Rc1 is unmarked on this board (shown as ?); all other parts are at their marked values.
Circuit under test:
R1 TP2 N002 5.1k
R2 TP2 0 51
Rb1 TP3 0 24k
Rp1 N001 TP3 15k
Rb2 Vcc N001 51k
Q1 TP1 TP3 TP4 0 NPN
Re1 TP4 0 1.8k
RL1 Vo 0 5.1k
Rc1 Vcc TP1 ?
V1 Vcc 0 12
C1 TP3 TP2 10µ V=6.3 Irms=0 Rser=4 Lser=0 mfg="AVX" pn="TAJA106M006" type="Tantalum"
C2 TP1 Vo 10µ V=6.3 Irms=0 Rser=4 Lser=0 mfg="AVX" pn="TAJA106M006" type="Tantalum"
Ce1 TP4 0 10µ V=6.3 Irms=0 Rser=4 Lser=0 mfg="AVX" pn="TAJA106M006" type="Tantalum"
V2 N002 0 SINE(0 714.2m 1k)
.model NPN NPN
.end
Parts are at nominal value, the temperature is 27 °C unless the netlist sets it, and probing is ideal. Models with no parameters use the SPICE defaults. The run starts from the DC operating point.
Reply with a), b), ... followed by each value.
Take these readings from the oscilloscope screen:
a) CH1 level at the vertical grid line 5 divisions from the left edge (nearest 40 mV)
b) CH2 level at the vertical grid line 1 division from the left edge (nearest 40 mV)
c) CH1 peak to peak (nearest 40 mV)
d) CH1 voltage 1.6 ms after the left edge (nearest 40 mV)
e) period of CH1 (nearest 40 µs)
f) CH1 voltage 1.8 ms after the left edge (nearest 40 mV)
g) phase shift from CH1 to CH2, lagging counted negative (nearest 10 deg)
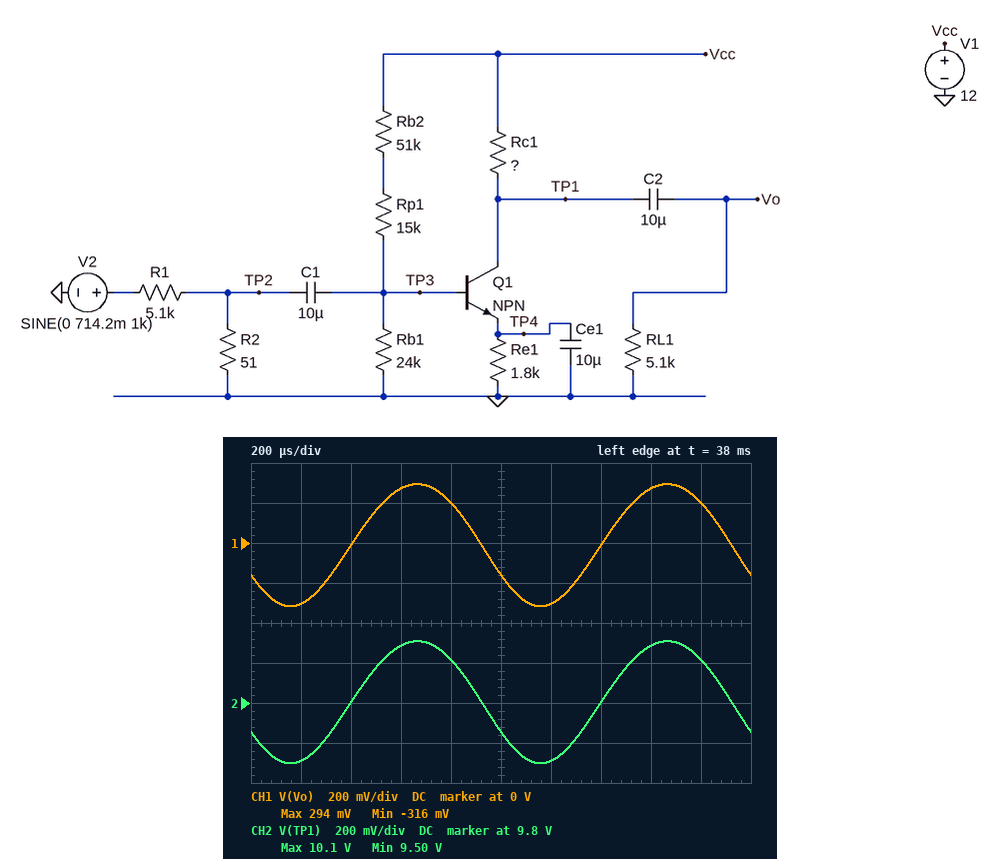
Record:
a) -160 mV
b) 9.52 V
c) 600 mV
d) 280 mV
e) 1.00 ms
f) 200 mV
g) 0 deg
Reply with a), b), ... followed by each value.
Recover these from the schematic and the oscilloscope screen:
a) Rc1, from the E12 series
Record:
a) 1.8 kΩ
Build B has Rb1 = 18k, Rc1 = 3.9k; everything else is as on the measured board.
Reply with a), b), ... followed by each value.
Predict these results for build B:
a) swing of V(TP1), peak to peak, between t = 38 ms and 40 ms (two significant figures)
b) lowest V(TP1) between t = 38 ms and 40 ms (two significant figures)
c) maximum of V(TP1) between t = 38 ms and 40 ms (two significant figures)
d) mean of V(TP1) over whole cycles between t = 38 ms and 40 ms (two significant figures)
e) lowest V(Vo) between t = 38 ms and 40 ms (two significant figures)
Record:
a) 850 mV
b) 8.0 V
c) 8.8 V
d) 8.4 V
e) -440 mV
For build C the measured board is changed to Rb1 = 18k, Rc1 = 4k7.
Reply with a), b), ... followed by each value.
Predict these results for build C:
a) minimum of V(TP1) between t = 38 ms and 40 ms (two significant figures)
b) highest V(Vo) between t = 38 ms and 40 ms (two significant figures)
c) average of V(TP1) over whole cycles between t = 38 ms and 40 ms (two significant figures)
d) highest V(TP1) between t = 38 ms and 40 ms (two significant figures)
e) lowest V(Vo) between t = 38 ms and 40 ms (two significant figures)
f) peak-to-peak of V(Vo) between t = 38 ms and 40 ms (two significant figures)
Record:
a) 7.2 V
b) 450 mV
c) 7.7 V
d) 8.1 V
e) -490 mV
f) 940 mV
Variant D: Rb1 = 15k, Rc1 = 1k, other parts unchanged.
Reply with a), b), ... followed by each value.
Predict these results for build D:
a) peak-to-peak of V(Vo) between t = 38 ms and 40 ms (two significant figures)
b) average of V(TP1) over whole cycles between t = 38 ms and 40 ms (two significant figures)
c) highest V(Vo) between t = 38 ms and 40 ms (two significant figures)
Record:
a) 280 mV
b) 11 V
c) 130 mV
